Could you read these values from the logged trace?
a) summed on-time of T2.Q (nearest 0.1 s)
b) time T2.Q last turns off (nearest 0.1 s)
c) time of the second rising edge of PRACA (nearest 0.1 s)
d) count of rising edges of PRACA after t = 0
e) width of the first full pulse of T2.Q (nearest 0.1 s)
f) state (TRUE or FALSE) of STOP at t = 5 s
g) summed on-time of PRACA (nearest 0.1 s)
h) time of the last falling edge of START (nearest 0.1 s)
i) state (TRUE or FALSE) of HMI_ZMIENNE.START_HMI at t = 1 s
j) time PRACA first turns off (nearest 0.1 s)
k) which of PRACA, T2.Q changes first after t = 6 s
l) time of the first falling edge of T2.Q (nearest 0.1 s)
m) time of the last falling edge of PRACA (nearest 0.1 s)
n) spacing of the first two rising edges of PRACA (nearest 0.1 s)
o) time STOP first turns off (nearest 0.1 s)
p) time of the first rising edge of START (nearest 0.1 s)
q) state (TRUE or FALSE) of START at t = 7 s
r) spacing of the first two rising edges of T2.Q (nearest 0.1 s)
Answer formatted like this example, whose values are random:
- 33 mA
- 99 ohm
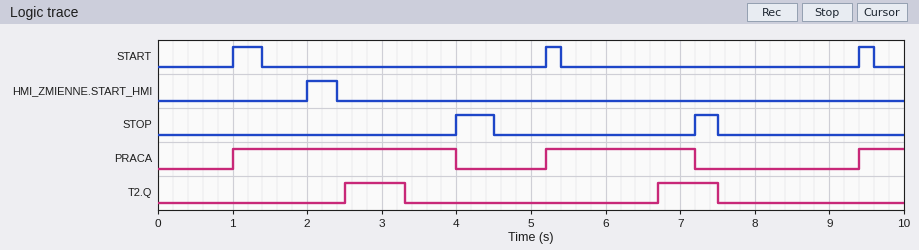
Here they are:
- 1.6 s
- 7.5 s
- 5.2 s
- 3
- 0.8 s
- FALSE
- 5.6 s
- 9.6 s
- FALSE
- 4.0 s
- T2.Q
- 3.3 s
- 7.2 s
- 4.2 s
- 4.5 s
- 1.0 s
- FALSE
- 4.2 s
